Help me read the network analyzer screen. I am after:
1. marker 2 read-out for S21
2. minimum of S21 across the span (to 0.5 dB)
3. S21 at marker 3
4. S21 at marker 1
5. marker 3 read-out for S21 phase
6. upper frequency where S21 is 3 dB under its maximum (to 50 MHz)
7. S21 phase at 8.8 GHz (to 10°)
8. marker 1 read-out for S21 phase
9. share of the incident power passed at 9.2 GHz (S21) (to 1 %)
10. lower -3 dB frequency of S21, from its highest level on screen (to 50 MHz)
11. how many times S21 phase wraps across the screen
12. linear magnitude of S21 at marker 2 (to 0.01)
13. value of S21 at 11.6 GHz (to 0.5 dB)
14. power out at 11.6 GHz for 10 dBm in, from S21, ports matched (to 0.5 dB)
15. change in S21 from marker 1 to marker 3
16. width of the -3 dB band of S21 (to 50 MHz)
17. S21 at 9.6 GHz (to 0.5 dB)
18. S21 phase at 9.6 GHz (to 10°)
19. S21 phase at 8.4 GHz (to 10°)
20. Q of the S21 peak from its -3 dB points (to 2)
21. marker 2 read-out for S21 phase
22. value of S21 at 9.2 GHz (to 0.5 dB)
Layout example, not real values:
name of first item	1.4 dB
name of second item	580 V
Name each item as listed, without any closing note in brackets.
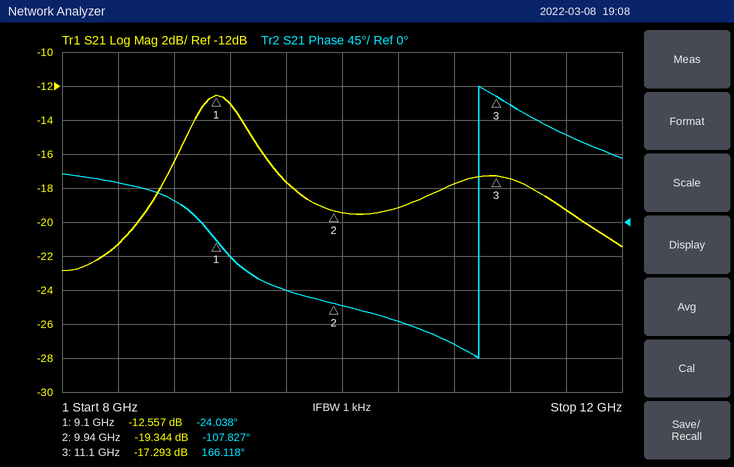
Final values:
marker 2 read-out for S21	-19.344 dB
minimum of S21 across the span	-23.0 dB
S21 at marker 3	-17.293 dB
S21 at marker 1	-12.557 dB
marker 3 read-out for S21 phase	166.118°
upper frequency where S21 is 3 dB under its maximum	9.40 GHz
S21 phase at 8.8 GHz	30°
marker 1 read-out for S21 phase	-24.038°
share of the incident power passed at 9.2 GHz (S21)	5 %
lower -3 dB frequency of S21, from its highest level on screen	8.85 GHz
how many times S21 phase wraps across the screen	1
linear magnitude of S21 at marker 2	0.11
value of S21 at 11.6 GHz	-19.5 dB
power out at 11.6 GHz for 10 dBm in, from S21, ports matched	-9.5 dBm
change in S21 from marker 1 to marker 3	-4.736 dB
width of the -3 dB band of S21	550 MHz
S21 at 9.6 GHz	-17.5 dB
S21 phase at 9.6 GHz	-90°
S21 phase at 8.4 GHz	50°
Q of the S21 peak from its -3 dB points	16
marker 2 read-out for S21 phase	-107.827°
value of S21 at 9.2 GHz	-13.0 dB
